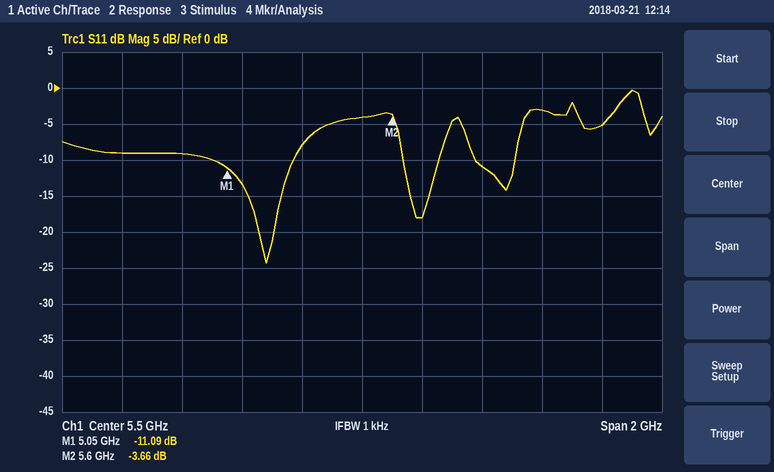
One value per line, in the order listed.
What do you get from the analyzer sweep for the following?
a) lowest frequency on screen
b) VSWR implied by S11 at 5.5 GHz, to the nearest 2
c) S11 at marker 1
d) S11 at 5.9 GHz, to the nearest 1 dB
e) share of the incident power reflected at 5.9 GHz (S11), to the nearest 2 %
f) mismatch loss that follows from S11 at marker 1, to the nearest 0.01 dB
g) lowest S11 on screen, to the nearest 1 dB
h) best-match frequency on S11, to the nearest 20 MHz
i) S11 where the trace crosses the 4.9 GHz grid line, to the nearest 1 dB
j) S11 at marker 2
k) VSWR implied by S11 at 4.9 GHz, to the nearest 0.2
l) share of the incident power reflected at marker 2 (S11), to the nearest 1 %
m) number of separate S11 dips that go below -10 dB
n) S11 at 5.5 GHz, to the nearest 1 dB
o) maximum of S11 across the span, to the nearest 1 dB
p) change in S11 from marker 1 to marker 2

4.5 GHz
4
-11.09 dB
-11 dB
8 %
0.35 dB
-24 dB
5.18 GHz
-9 dB
-3.66 dB
2.0
43 %
3
-4 dB
0 dB
7.43 dB
